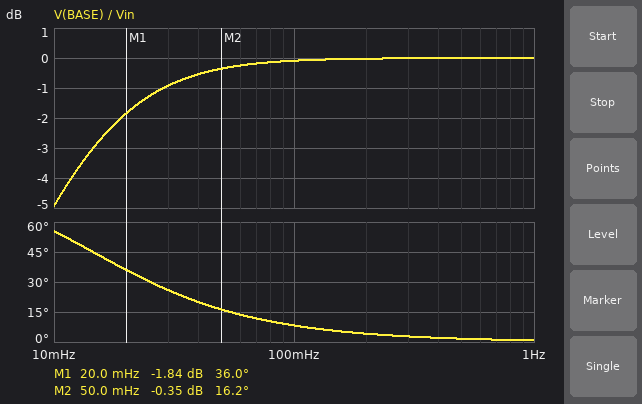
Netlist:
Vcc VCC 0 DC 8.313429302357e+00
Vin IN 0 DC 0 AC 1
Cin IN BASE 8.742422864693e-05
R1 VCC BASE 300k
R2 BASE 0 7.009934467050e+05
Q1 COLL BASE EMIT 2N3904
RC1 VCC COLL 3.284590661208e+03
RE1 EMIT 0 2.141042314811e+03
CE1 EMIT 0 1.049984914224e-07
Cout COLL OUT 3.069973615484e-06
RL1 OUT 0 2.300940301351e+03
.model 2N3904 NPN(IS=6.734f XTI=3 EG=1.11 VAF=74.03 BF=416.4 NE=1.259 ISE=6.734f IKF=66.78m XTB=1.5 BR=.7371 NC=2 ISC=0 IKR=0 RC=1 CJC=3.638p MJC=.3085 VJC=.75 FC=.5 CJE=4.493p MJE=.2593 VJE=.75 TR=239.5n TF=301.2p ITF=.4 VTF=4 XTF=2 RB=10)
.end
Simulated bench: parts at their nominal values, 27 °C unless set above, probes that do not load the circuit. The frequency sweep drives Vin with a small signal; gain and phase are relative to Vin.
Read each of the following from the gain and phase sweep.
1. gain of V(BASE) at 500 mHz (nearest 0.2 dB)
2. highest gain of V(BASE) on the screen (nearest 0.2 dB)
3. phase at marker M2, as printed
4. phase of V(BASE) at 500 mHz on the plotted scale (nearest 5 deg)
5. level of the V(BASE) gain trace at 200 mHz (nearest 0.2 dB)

0 dB
0 dB
16.2 deg
0 deg
0 dB
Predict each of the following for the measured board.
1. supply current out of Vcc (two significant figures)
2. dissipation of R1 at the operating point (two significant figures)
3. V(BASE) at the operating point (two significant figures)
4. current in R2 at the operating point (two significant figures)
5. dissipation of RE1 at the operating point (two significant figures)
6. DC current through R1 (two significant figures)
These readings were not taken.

1.4 mA
71 µW
3.7 V
5.3 µA
4.3 mW
15 µA
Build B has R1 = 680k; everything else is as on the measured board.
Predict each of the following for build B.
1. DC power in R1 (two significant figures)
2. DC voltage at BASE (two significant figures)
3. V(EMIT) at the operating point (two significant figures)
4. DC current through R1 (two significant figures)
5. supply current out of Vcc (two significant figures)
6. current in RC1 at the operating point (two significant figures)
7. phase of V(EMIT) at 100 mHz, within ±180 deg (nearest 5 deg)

54 µW
2.3 V
1.6 V
8.9 µA
760 µA
750 µA
5 deg
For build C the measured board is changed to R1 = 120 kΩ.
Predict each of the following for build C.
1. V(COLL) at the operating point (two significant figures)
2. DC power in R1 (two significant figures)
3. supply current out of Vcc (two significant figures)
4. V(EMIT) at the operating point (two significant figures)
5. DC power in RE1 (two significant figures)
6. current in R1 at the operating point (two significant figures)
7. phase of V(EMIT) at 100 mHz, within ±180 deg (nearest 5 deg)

3.4 V
160 µW
1.5 mA
3.3 V
5.0 mW
36 µA
85 deg
